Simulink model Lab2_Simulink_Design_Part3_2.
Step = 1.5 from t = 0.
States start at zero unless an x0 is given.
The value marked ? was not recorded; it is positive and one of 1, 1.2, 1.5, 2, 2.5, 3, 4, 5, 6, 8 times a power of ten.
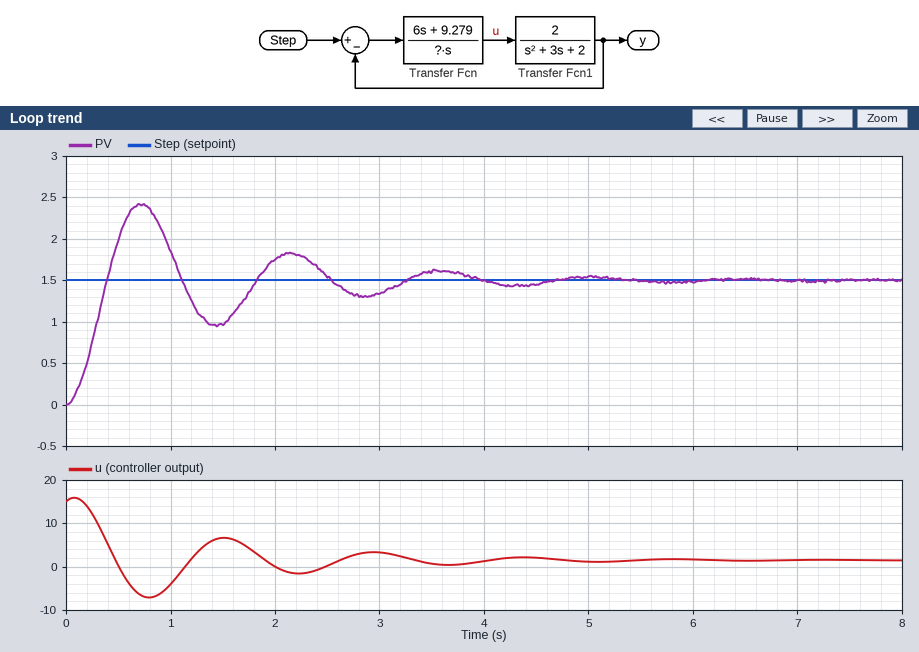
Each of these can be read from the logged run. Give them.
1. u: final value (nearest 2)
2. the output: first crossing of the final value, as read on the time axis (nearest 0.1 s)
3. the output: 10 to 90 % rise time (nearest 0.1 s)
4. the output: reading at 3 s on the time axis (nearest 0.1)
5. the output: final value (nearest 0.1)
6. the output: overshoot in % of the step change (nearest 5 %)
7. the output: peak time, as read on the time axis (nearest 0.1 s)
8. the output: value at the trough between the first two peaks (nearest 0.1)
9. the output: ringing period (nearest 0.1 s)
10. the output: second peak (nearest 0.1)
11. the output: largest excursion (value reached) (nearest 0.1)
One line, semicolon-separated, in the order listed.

2; 0.4 s; 0.3 s; 1.3; 1.5; 60 %; 0.7 s; 1.0; 1.4 s; 1.8; 2.4
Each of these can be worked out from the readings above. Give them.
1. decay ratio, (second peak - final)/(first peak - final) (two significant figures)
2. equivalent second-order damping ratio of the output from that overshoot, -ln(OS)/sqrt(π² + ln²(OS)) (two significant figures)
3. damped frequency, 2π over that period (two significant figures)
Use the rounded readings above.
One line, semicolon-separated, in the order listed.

0.33; 0.16; 4.5 rad/s
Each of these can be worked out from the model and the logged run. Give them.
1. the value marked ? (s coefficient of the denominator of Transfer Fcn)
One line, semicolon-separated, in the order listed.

0.6
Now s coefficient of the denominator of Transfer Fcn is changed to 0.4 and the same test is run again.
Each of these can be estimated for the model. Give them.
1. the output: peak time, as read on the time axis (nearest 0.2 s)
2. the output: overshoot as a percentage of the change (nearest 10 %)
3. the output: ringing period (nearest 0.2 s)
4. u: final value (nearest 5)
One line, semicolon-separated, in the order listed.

0.6 s; 70 %; 1.2 s; 0
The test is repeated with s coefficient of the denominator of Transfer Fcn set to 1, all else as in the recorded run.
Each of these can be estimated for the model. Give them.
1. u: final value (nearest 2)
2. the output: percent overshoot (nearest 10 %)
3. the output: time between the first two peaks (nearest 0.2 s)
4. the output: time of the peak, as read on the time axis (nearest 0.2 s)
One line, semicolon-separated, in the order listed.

2; 50 %; 1.8 s; 1.0 s
